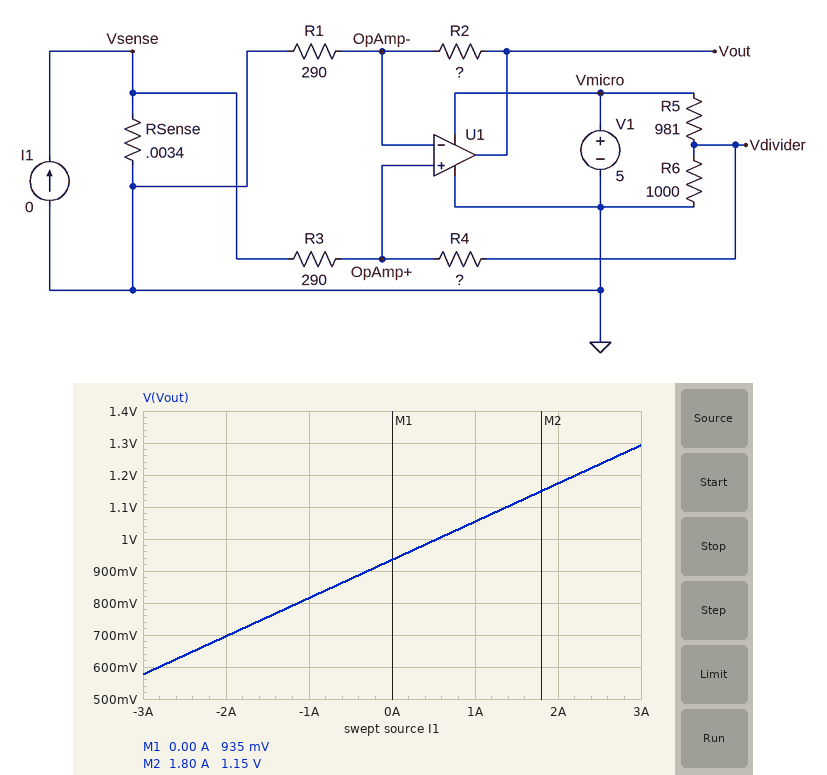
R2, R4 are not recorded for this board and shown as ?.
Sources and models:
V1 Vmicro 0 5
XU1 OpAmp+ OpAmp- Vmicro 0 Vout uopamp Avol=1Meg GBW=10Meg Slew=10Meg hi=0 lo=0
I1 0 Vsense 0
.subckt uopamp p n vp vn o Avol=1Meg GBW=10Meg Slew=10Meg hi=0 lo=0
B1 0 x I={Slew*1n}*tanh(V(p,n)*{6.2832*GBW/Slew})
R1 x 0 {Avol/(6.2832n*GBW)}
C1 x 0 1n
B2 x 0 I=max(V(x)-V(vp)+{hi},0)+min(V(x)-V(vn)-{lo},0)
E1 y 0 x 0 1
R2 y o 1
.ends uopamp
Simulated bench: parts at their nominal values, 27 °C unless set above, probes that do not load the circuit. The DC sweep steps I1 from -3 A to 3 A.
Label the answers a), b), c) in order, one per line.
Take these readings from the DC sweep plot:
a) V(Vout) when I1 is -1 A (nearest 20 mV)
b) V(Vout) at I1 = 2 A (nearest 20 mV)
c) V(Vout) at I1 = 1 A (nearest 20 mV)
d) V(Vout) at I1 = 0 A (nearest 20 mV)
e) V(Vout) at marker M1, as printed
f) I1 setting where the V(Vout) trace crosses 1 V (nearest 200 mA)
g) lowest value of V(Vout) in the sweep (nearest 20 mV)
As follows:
a) 820 mV
b) 1.18 V
c) 1.06 V
d) 940 mV
e) 935 mV
f) 600 mA
g) 580 mV
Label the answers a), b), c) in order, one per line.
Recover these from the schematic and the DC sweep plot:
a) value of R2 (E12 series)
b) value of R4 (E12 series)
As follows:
a) 10 kΩ
b) 27 kΩ
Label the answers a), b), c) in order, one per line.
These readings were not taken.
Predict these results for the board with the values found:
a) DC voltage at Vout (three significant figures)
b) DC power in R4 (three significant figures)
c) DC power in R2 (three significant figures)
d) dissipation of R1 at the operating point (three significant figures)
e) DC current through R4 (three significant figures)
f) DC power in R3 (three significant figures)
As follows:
a) 935 mV
b) 223 µW
c) 82.5 µW
d) 2.39 µW
e) 90.8 µA
f) 2.39 µW
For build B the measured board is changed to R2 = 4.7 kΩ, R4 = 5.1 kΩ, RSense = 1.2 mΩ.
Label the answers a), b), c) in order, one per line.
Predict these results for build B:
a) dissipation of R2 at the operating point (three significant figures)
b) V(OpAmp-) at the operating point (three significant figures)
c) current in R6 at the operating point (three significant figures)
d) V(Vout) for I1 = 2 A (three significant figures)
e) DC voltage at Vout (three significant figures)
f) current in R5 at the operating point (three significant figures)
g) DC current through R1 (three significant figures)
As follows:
a) 864 µW
b) 124 mV
c) 2.31 mA
d) 2.18 V
e) 2.14 V
f) 2.74 mA
g) 429 µA
